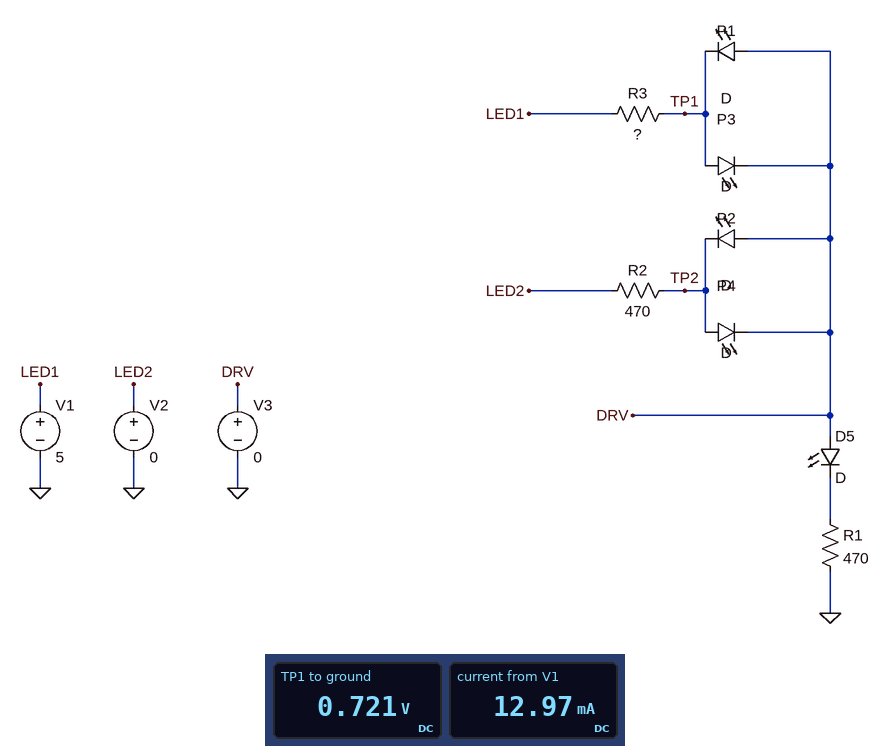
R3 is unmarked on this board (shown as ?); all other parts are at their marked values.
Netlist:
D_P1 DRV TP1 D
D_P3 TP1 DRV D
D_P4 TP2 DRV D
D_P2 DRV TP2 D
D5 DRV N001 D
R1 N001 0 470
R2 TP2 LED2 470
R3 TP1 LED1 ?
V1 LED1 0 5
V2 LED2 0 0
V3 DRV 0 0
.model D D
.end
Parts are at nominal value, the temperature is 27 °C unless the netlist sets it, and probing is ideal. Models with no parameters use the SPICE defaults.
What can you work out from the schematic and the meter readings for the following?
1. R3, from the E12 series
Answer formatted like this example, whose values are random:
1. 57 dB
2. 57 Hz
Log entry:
1. 330 Ω
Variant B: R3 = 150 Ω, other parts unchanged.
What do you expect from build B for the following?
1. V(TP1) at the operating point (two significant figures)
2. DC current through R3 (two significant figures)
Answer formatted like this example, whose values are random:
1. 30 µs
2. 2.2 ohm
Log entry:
1. 740 mV
2. 28 mA
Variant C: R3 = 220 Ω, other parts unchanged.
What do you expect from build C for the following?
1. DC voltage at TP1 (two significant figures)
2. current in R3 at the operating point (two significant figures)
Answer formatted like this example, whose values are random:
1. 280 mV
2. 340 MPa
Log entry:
1. 730 mV
2. 19 mA
